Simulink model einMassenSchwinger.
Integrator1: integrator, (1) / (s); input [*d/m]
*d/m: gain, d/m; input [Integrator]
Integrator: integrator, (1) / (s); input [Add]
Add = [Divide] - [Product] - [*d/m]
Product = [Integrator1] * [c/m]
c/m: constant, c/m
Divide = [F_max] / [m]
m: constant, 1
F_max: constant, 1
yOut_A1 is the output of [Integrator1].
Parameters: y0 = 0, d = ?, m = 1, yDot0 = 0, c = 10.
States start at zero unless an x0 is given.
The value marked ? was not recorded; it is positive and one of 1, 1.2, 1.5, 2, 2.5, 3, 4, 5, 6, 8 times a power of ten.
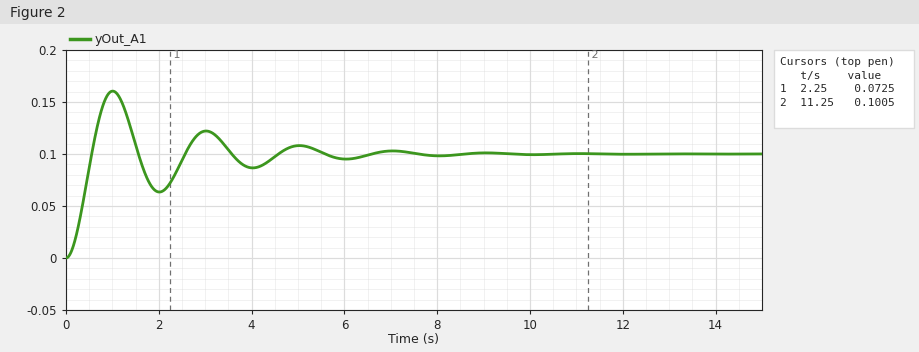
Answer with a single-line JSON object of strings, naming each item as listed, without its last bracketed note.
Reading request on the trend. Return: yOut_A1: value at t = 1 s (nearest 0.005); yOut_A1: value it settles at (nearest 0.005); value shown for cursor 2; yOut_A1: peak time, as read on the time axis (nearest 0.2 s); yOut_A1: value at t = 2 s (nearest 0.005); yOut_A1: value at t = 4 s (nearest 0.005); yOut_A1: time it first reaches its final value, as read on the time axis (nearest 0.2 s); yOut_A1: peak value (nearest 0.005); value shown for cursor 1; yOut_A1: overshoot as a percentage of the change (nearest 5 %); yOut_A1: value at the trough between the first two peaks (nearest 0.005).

{"yOut_A1: value at t = 1 s": "0.160", "yOut_A1: value it settles at": "0.100", "value shown for cursor 2": "0.1005", "yOut_A1: peak time, as read on the time axis": "1.0 s", "yOut_A1: value at t = 2 s": "0.065", "yOut_A1: value at t = 4 s": "0.085", "yOut_A1: time it first reaches its final value, as read on the time axis": "0.6 s", "yOut_A1: peak value": "0.160", "value shown for cursor 1": "0.0725", "yOut_A1: overshoot as a percentage of the change": "60 %", "yOut_A1: value at the trough between the first two peaks": "0.065"}
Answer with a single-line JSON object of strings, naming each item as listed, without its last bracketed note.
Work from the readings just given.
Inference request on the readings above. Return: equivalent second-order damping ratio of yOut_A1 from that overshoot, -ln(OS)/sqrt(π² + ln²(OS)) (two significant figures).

{"equivalent second-order damping ratio of yOut_A1 from that overshoot, -ln(OS)/sqrt(π² + ln²(OS))": "0.16"}
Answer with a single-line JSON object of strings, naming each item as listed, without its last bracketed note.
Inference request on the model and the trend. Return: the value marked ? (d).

{"the value marked ?": "1"}
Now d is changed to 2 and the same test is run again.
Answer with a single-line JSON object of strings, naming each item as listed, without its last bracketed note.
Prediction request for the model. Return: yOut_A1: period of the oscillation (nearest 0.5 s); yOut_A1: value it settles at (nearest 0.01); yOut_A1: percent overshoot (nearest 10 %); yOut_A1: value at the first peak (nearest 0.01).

{"yOut_A1: period of the oscillation": "1.5 s", "yOut_A1: value it settles at": "0.10", "yOut_A1: percent overshoot": "50 %", "yOut_A1: value at the first peak": "0.15"}
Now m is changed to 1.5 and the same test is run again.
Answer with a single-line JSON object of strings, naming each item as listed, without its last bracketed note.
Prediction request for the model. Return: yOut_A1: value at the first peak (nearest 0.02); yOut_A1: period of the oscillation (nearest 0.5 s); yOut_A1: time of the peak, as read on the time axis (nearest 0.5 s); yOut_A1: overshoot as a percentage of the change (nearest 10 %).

{"yOut_A1: value at the first peak": "0.24", "yOut_A1: period of the oscillation": "3.0 s", "yOut_A1: time of the peak, as read on the time axis": "1.5 s", "yOut_A1: overshoot as a percentage of the change": "60 %"}
